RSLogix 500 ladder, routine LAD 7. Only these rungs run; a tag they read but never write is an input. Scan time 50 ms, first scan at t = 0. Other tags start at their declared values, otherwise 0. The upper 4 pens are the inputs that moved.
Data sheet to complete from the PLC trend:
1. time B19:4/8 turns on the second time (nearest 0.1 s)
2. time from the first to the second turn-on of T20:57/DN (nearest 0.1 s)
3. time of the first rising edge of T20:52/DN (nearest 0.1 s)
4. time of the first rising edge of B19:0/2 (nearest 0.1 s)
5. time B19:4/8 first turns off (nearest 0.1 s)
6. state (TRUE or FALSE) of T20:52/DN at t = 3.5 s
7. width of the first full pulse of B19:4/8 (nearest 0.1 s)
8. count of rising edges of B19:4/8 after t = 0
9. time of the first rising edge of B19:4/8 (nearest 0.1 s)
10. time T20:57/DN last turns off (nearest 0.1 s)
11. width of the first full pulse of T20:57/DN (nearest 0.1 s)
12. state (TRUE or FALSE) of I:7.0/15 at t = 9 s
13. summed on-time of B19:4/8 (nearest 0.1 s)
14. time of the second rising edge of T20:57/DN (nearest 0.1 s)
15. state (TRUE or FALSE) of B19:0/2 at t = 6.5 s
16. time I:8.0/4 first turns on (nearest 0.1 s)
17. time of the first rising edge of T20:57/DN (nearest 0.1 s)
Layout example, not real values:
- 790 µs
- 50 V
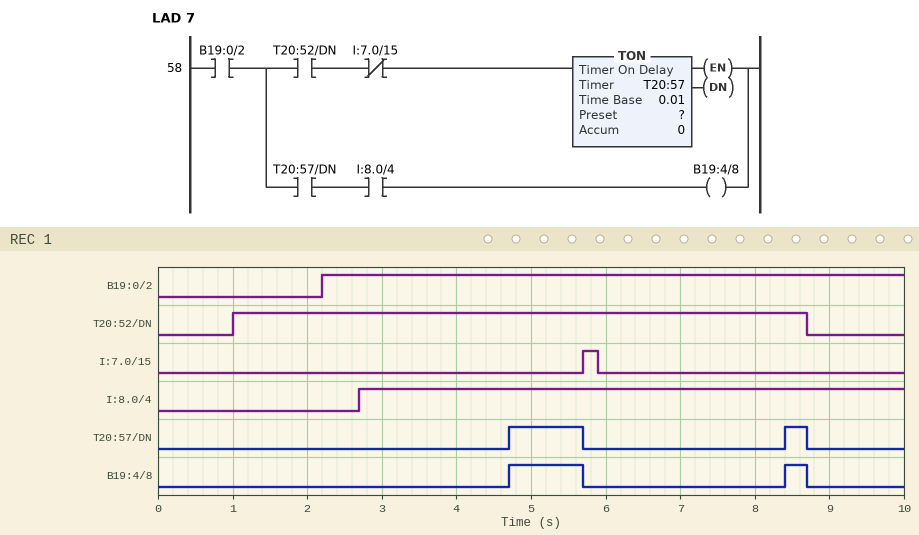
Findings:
- 8.4 s
- 3.7 s
- 1.0 s
- 2.2 s
- 5.7 s
- TRUE
- 1.0 s
- 2
- 4.7 s
- 8.7 s
- 1.0 s
- FALSE
- 1.3 s
- 8.4 s
- TRUE
- 2.7 s
- 4.7 s
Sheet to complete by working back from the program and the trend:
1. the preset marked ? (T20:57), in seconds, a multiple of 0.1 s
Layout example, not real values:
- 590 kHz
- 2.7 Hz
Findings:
- 2.5 s
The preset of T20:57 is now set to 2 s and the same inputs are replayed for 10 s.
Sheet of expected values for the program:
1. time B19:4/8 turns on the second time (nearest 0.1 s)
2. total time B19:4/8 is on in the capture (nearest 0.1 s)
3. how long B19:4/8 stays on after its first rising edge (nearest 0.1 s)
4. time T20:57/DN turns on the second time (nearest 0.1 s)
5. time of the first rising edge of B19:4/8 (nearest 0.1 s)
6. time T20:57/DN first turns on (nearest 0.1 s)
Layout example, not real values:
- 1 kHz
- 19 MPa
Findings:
- 7.9 s
- 2.3 s
- 1.5 s
- 7.9 s
- 4.2 s
- 4.2 s
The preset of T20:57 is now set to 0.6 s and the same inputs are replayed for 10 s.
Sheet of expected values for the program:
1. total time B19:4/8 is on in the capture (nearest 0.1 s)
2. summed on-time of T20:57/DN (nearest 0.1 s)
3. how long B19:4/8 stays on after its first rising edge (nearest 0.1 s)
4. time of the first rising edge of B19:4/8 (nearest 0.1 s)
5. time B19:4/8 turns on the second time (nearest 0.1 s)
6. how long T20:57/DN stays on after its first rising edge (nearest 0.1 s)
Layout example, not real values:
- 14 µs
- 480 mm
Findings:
- 5.1 s
- 5.1 s
- 2.9 s
- 2.8 s
- 6.5 s
- 2.9 s
